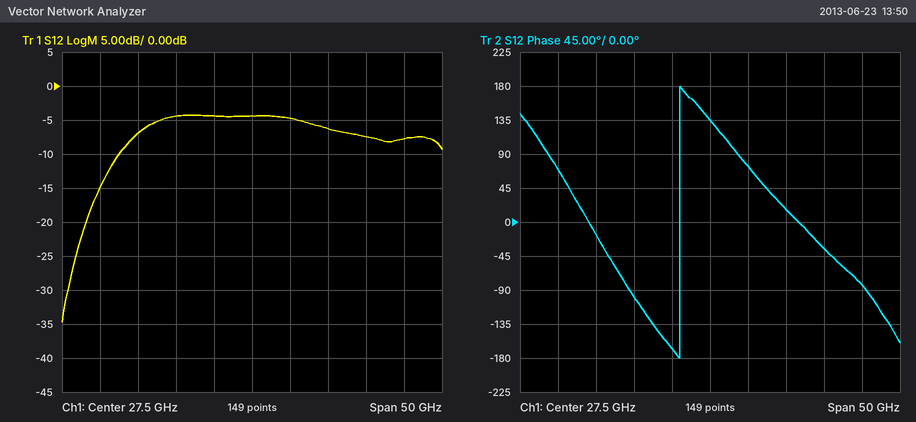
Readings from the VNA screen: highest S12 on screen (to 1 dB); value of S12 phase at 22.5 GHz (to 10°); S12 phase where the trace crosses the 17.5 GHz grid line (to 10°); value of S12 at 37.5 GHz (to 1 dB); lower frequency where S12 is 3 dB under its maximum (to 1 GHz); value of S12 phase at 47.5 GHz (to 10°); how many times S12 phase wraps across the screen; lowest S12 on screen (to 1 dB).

-4 dB
-170°
-100°
-6 dB
12 GHz
-80°
1
-35 dB
